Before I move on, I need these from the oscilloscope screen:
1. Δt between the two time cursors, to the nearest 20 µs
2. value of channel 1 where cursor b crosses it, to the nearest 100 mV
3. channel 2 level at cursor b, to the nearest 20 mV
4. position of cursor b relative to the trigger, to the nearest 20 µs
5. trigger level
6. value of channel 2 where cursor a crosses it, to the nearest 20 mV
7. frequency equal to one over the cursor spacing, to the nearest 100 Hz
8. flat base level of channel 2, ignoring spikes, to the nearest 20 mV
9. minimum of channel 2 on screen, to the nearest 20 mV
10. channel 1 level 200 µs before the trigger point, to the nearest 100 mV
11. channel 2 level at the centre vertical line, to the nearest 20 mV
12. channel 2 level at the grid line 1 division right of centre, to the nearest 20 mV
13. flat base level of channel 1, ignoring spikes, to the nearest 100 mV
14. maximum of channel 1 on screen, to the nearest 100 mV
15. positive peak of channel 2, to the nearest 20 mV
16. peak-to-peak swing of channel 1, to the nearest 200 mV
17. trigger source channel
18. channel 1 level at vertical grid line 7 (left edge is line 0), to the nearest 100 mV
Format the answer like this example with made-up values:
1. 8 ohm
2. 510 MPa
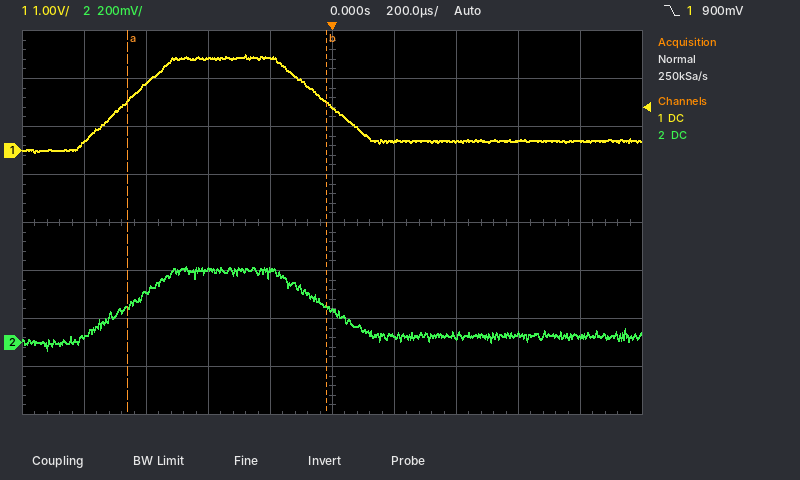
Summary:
1. 640 µs
2. 1.0 V
3. 140 mV
4. -20 µs
5. 900 mV
6. 160 mV
7. 1.6 kHz
8. 20 mV
9. -40 mV
10. 1.9 V
11. 140 mV
12. 20 mV
13. 200 mV
14. 2.0 V
15. 320 mV
16. 2.0 V
17. channel 1
18. 200 mV
